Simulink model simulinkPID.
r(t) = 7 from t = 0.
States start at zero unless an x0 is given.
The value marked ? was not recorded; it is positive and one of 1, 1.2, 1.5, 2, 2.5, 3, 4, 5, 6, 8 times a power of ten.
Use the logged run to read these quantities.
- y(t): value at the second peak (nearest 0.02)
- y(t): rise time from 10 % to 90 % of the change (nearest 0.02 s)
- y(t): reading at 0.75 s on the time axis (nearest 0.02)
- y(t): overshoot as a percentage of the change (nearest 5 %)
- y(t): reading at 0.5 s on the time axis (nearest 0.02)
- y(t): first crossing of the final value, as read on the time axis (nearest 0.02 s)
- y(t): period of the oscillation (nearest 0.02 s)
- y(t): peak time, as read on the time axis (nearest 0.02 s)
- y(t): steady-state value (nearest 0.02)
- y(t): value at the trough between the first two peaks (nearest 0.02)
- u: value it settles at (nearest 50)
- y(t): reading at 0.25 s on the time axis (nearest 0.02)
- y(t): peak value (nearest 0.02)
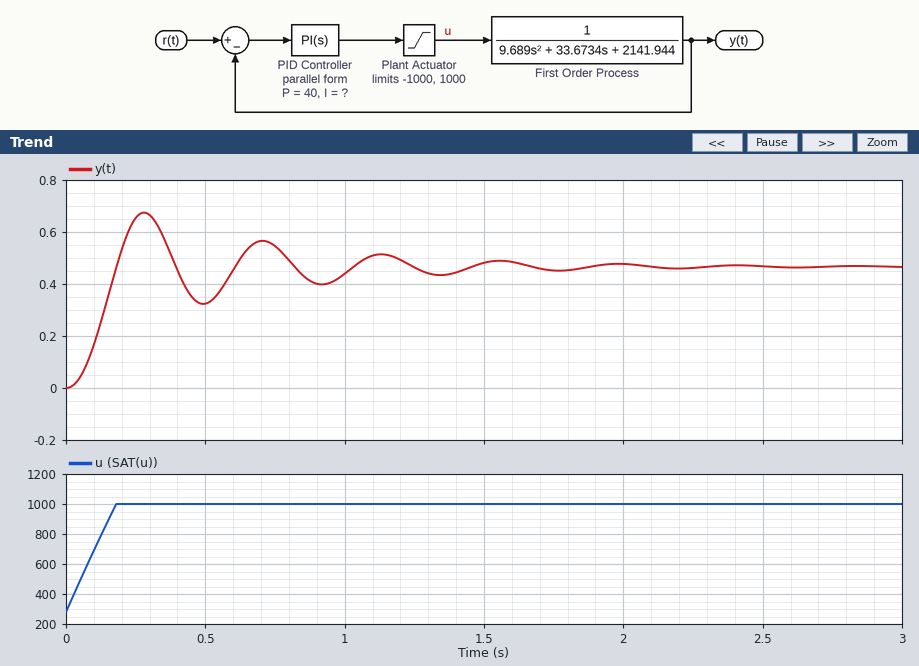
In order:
0.56
0.12 s
0.54
45 %
0.32
0.18 s
0.42 s
0.28 s
0.46
0.32
1000
0.66
0.68
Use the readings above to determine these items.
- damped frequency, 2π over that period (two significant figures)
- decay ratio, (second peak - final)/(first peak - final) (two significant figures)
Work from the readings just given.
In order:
15 rad/s
0.45
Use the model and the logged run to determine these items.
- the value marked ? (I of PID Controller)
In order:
600
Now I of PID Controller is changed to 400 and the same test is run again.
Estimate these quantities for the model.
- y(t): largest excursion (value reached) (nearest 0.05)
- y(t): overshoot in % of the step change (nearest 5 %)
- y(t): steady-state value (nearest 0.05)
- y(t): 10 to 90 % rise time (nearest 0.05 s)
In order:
0.55
20 %
0.45
0.15 s
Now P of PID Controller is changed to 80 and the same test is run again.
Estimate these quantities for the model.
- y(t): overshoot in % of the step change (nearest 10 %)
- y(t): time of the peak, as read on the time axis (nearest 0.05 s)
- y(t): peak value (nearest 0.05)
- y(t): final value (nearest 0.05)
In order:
60 %
0.25 s
0.75
0.45
